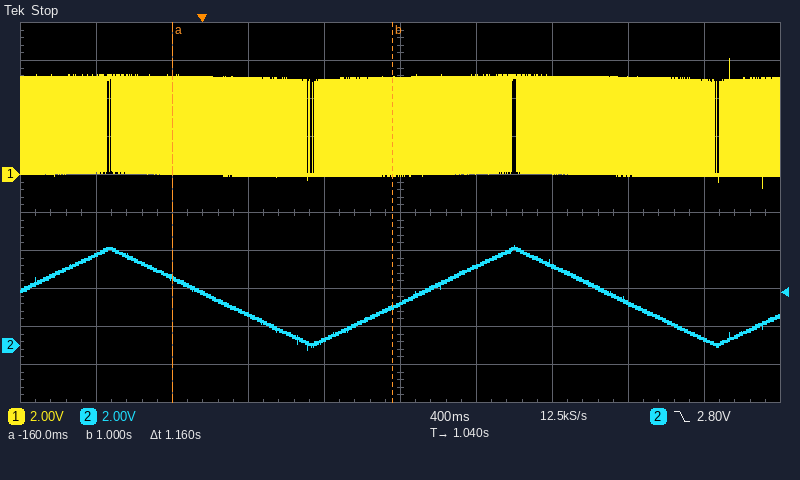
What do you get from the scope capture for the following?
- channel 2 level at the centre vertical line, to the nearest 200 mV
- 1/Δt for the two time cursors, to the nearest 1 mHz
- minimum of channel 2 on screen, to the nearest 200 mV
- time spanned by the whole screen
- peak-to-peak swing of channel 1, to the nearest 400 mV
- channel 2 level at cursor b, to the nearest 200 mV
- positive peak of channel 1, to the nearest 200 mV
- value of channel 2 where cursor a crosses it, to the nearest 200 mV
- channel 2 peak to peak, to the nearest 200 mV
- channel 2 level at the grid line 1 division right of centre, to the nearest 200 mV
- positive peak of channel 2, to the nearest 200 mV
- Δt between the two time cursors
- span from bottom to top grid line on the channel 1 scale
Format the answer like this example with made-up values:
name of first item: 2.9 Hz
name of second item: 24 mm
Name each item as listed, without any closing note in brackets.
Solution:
channel 2 level at the centre vertical line, to the nearest 200 mV: 2.2 V
1/Δt for the two time cursors, to the nearest 1 mHz: 862 mHz
minimum of channel 2 on screen, to the nearest 200 mV: -200 mV
time spanned by the whole screen: 4 s
peak-to-peak swing of channel 1, to the nearest 400 mV: 6.8 V
channel 2 level at cursor b, to the nearest 200 mV: 2.0 V
positive peak of channel 1, to the nearest 200 mV: 6.2 V
value of channel 2 where cursor a crosses it, to the nearest 200 mV: 3.6 V
channel 2 peak to peak, to the nearest 200 mV: 5.4 V
channel 2 level at the grid line 1 division right of centre, to the nearest 200 mV: 4.2 V
positive peak of channel 2, to the nearest 200 mV: 5.2 V
Δt between the two time cursors: 1.16 s
span from bottom to top grid line on the channel 1 scale: 20 V
